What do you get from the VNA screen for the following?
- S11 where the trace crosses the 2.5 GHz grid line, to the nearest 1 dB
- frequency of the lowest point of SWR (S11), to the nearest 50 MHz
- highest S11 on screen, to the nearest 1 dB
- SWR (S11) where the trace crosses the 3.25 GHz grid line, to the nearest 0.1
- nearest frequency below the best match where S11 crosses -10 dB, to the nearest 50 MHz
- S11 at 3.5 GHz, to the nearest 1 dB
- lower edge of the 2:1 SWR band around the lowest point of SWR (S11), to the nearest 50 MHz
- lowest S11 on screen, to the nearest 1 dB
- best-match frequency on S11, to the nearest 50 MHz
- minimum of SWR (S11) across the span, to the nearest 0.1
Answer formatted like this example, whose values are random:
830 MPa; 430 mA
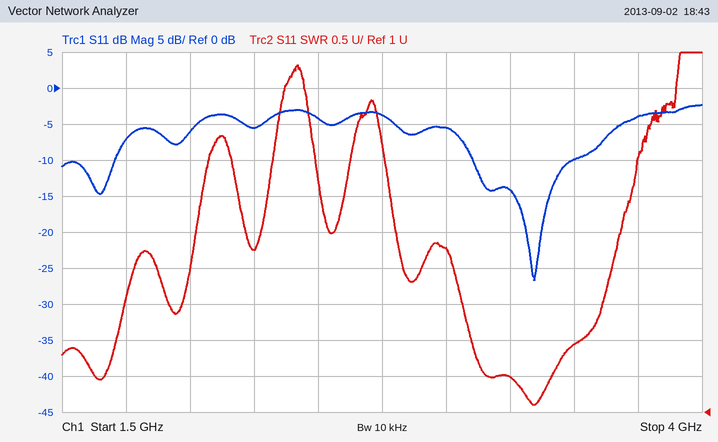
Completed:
-4 dB; 3.35 GHz; -2 dB; 1.5; 3.10 GHz; -10 dB; 3.10 GHz; -27 dB; 3.35 GHz; 1.1
